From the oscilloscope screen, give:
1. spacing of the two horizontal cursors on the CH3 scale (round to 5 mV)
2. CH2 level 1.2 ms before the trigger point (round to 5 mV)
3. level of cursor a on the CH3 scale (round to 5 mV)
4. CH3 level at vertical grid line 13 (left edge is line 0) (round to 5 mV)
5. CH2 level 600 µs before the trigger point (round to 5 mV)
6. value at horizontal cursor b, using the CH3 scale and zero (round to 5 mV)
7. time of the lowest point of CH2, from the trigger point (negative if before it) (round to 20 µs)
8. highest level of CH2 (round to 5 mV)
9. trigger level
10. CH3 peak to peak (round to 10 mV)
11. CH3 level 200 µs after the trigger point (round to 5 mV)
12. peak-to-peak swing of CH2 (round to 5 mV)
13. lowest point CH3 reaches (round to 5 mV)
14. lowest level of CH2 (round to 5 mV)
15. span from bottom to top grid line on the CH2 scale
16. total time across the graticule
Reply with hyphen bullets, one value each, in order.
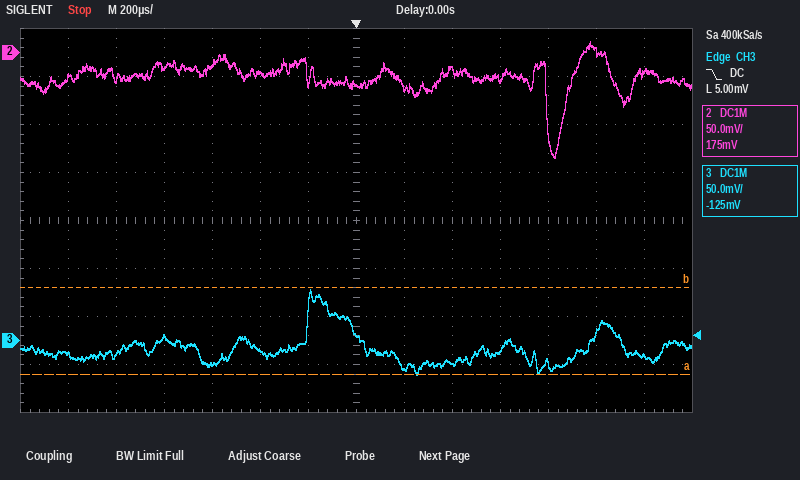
- 90 mV
- -25 mV
- -35 mV
- -15 mV
- -10 mV
- 55 mV
- +820 µs
- 10 mV
- 5.00 mV
- 90 mV
- -30 mV
- 120 mV
- -35 mV
- -110 mV
- 400 mV
- 2.8 ms
